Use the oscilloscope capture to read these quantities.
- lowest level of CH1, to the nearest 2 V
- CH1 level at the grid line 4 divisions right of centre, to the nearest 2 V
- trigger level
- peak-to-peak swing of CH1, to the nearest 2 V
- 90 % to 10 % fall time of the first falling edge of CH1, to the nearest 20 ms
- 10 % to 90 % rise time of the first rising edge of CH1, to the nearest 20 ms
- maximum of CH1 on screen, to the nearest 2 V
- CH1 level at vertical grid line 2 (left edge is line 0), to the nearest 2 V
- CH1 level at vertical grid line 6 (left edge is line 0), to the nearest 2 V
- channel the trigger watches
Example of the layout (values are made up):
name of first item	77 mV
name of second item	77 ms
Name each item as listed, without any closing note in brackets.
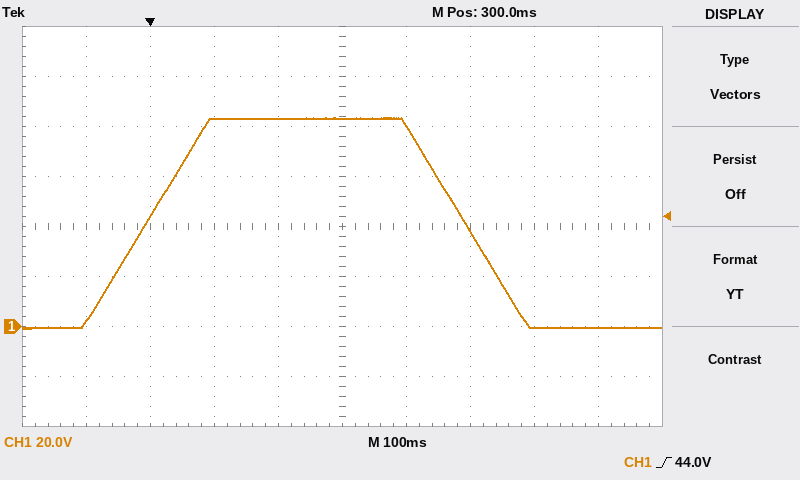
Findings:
lowest level of CH1, to the nearest 2 V	0 V
CH1 level at the grid line 4 divisions right of centre, to the nearest 2 V	0 V
trigger level	44.0 V
peak-to-peak swing of CH1, to the nearest 2 V	84 V
90 % to 10 % fall time of the first falling edge of CH1, to the nearest 20 ms	160 ms
10 % to 90 % rise time of the first rising edge of CH1, to the nearest 20 ms	160 ms
maximum of CH1 on screen, to the nearest 2 V	84 V
CH1 level at vertical grid line 2 (left edge is line 0), to the nearest 2 V	44 V
CH1 level at vertical grid line 6 (left edge is line 0), to the nearest 2 V	80 V
channel the trigger watches	CH1
